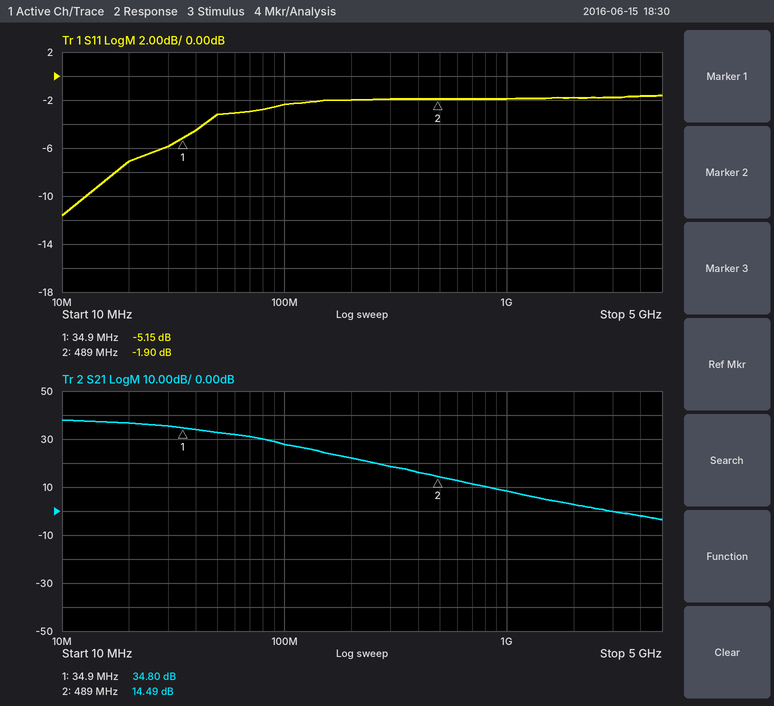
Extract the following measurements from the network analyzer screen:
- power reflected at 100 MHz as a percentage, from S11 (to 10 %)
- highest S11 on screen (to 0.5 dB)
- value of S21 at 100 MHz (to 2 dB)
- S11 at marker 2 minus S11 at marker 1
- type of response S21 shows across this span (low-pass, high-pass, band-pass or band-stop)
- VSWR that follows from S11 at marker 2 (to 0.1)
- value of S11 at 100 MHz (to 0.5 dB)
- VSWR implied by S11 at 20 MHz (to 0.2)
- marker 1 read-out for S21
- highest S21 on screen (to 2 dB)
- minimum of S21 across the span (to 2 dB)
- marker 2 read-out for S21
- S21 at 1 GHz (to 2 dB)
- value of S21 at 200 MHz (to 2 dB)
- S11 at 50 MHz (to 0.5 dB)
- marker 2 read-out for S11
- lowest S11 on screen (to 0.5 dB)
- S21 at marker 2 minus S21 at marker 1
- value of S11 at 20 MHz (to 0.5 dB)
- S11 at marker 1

60 %
-1.5 dB
28 dB
3.25 dB
low-pass
9.2
-2.5 dB
2.6
34.80 dB
38 dB
-4 dB
14.49 dB
8 dB
22 dB
-3.0 dB
-1.90 dB
-11.5 dB
-20.31 dB
-7.0 dB
-5.15 dB
